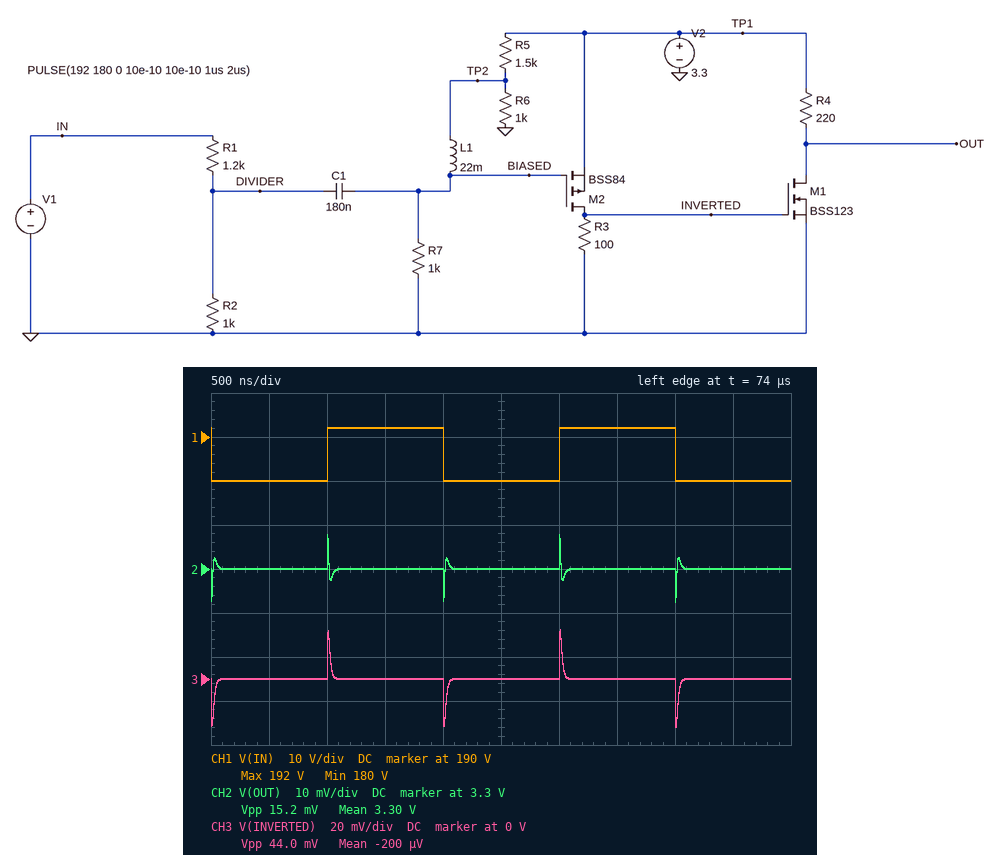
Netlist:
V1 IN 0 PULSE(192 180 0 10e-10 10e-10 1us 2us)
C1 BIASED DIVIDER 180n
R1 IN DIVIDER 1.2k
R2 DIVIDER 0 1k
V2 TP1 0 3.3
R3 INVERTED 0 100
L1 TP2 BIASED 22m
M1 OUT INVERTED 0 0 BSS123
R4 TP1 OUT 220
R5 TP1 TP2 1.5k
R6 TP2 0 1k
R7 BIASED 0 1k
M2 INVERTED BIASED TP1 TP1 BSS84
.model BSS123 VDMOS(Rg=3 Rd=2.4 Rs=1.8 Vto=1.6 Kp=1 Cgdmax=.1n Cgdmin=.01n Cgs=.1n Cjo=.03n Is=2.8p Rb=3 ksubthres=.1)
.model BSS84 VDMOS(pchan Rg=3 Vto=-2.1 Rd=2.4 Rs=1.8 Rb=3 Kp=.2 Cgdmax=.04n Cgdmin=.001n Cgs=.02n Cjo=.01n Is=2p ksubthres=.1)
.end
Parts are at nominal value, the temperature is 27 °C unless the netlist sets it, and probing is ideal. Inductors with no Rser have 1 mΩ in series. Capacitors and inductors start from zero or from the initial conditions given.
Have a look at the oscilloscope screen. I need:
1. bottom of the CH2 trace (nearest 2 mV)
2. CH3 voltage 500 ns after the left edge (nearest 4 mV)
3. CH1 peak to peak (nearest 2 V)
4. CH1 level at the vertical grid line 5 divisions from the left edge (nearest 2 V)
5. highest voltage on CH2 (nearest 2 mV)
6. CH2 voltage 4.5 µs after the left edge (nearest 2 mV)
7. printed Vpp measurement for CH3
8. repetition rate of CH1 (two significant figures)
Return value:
3.292 V
0 V
12 V
180 V
3.308 V
3.300 V
44.0 mV
500 kHz
